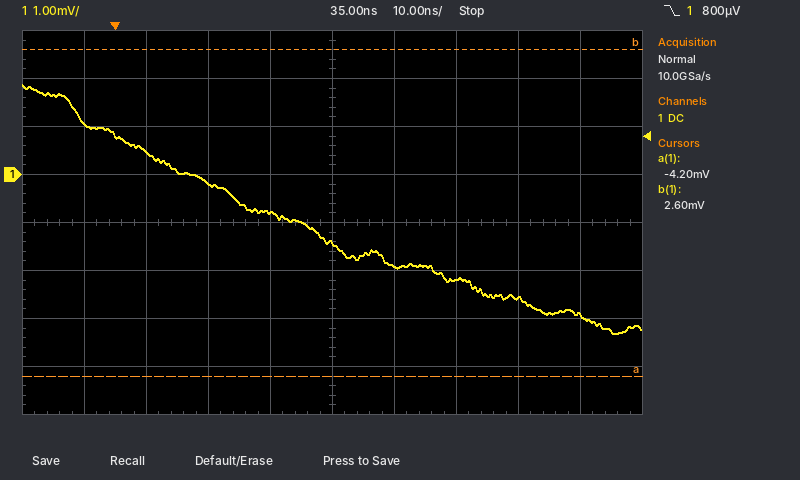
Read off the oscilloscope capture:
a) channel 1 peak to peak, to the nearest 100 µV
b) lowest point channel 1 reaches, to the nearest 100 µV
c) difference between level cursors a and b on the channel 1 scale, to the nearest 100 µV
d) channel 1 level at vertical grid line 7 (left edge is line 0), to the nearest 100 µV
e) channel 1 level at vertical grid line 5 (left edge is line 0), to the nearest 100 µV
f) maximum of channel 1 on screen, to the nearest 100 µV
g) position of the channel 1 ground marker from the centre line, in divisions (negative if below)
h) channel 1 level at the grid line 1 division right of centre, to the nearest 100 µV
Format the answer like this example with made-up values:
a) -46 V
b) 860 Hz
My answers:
a) 5.2 mV
b) -3.3 mV
c) 6.8 mV
d) -2.2 mV
e) -1.4 mV
f) 1.9 mV
g) +1.0 div
h) -1.9 mV
